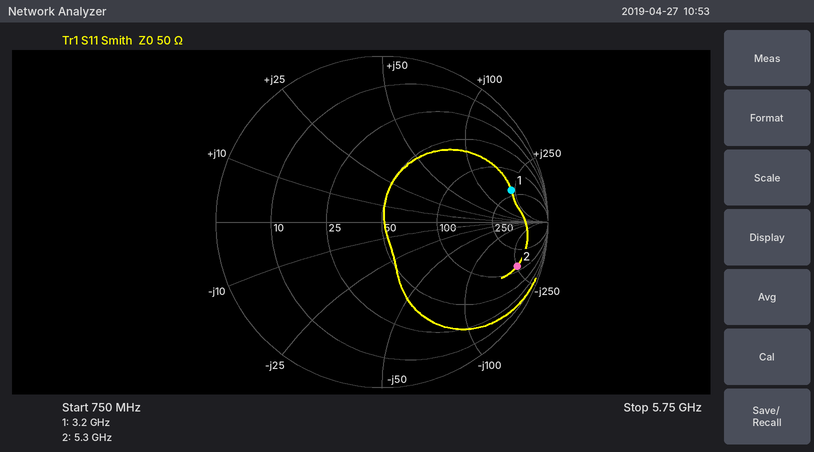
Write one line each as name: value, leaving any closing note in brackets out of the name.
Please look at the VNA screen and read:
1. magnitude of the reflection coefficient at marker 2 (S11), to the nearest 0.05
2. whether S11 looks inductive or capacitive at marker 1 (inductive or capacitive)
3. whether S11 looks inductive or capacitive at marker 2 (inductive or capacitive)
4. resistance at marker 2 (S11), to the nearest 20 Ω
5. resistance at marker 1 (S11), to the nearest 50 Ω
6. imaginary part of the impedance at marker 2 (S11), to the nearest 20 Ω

magnitude of the reflection coefficient at marker 2 (S11), to the nearest 0.05: 0.85
whether S11 looks inductive or capacitive at marker 1: inductive
whether S11 looks inductive or capacitive at marker 2: capacitive
resistance at marker 2 (S11), to the nearest 20 Ω: 120 Ω
resistance at marker 1 (S11), to the nearest 50 Ω: 200 Ω
imaginary part of the impedance at marker 2 (S11), to the nearest 20 Ω: -260 Ω
